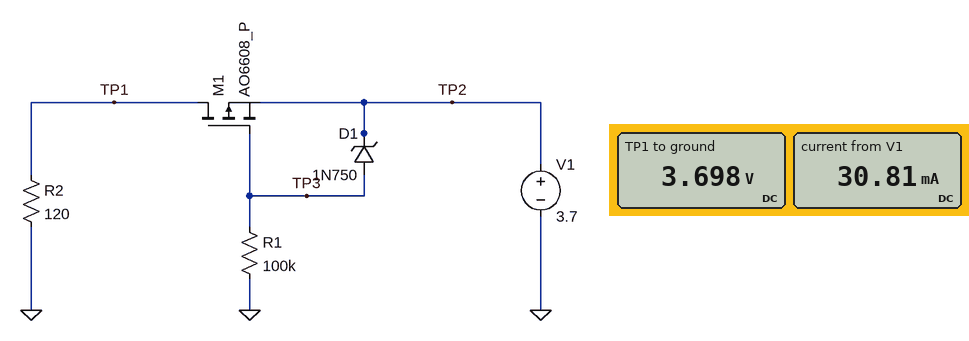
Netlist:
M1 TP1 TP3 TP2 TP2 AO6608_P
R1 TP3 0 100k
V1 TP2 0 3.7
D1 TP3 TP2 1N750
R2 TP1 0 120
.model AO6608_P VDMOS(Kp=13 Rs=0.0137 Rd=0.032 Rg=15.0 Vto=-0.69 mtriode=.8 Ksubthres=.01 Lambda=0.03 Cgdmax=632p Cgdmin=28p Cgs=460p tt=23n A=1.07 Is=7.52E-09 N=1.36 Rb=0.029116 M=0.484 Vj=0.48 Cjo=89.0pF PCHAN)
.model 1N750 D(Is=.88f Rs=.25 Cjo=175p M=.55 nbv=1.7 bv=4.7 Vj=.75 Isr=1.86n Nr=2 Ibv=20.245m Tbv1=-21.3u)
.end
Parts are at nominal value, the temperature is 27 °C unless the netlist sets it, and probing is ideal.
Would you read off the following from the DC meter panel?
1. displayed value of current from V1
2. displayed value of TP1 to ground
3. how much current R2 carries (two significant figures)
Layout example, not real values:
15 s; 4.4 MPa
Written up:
30.81 mA; 3.698 V; 31 mA
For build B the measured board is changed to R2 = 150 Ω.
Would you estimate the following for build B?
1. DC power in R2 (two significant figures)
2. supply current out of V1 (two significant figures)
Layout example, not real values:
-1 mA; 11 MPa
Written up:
91 mW; 25 mA
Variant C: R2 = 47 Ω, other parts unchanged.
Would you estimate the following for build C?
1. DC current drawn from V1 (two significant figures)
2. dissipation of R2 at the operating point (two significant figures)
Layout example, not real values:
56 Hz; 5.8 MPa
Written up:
79 mA; 290 mW
